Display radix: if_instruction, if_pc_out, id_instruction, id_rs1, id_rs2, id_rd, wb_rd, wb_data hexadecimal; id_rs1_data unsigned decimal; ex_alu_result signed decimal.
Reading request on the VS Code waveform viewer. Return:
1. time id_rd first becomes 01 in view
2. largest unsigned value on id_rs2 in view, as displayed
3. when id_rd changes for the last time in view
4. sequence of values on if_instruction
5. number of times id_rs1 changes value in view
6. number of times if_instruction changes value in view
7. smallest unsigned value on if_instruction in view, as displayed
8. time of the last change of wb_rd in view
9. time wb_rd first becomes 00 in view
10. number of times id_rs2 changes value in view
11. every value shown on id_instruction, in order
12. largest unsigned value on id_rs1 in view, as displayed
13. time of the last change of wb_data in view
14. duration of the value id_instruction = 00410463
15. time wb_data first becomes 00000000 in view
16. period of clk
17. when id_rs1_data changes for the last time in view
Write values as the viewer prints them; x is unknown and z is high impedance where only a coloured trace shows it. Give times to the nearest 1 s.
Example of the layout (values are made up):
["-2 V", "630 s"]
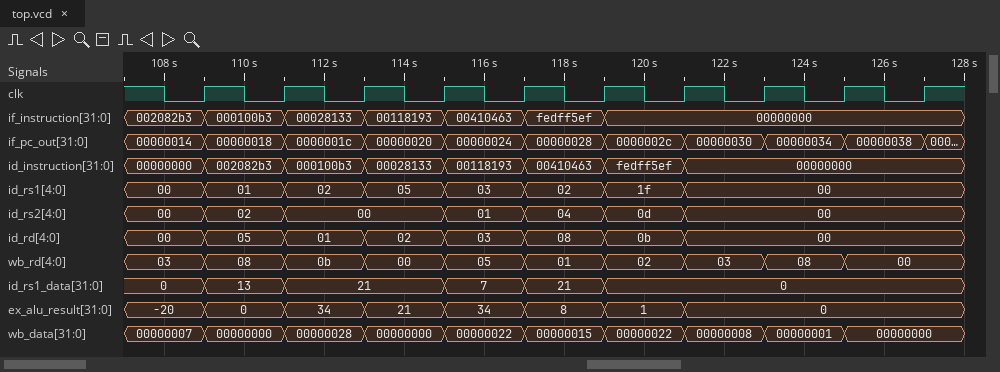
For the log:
["111 s", "0d", "121 s", "002082b3, 000100b3, 00028133, 00118193, 00410463, fedff5ef, 00000000", "7", "6", "00000000", "125 s", "113 s", "6", "00000000, 002082b3, 000100b3, 00028133, 00118193, 00410463, fedff5ef, 00000000", "1f", "125 s", "2 s", "109 s", "2 s", "119 s"]
